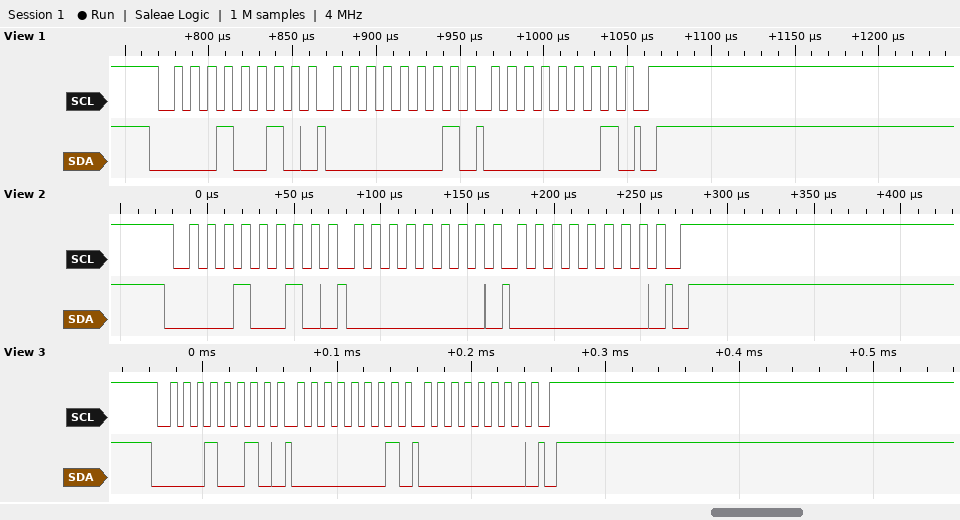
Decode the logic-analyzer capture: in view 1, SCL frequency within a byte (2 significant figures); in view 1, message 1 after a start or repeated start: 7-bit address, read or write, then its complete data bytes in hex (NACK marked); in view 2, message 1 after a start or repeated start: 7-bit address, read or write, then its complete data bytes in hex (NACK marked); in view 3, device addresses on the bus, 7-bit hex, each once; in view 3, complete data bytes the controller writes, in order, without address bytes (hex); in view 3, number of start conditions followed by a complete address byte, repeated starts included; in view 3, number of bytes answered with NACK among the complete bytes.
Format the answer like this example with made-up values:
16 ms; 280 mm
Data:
100 kHz; 0x09 write: 01 01; 0x09 write: 00 00; 0x09; 01 00; 1; 0
